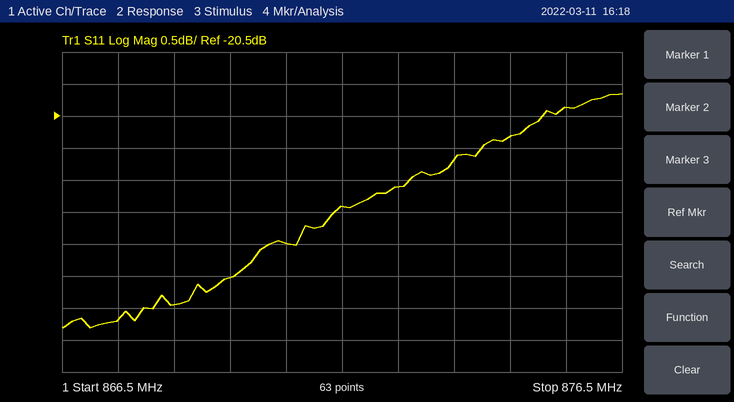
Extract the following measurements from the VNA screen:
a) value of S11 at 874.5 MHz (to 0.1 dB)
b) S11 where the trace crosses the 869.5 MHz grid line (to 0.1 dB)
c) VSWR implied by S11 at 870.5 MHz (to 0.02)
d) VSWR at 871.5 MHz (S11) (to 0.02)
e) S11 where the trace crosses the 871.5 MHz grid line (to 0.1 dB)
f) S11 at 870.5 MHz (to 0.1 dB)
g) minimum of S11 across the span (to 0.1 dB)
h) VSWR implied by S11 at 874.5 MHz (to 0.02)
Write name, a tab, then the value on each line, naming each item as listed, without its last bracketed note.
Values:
value of S11 at 874.5 MHz	-20.8 dB
S11 where the trace crosses the 869.5 MHz grid line	-23.0 dB
VSWR implied by S11 at 870.5 MHz	1.16
VSWR at 871.5 MHz (S11)	1.18
S11 where the trace crosses the 871.5 MHz grid line	-21.9 dB
S11 at 870.5 MHz	-22.5 dB
minimum of S11 across the span	-23.8 dB
VSWR implied by S11 at 874.5 MHz	1.20
